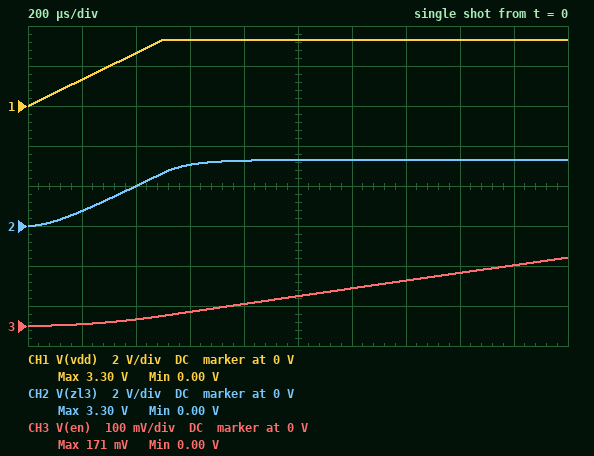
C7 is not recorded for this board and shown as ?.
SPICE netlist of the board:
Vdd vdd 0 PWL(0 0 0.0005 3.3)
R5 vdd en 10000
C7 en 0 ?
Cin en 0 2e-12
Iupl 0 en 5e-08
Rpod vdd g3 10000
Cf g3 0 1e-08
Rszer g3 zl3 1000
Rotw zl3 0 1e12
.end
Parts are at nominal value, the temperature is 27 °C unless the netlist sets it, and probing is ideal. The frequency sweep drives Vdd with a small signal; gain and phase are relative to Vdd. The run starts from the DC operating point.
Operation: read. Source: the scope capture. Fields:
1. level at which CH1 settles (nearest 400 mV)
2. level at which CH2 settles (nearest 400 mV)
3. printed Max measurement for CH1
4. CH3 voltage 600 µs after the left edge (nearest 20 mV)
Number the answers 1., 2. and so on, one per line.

1. 3.2 V
2. 3.2 V
3. 3.30 V
4. 40 mV
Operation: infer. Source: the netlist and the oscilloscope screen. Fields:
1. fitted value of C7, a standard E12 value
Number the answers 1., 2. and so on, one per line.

1. 3.3 µF
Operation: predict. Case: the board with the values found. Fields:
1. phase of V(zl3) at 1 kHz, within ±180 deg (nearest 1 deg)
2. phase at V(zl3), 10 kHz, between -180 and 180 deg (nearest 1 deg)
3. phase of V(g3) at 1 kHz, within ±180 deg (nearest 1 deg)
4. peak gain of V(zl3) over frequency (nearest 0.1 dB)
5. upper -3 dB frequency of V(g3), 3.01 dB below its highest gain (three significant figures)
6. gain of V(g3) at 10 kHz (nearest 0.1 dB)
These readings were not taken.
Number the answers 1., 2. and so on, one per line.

1. -32 deg
2. -81 deg
3. -32 deg
4. 0 dB
5. 1.59 kHz
6. -16.1 dB
